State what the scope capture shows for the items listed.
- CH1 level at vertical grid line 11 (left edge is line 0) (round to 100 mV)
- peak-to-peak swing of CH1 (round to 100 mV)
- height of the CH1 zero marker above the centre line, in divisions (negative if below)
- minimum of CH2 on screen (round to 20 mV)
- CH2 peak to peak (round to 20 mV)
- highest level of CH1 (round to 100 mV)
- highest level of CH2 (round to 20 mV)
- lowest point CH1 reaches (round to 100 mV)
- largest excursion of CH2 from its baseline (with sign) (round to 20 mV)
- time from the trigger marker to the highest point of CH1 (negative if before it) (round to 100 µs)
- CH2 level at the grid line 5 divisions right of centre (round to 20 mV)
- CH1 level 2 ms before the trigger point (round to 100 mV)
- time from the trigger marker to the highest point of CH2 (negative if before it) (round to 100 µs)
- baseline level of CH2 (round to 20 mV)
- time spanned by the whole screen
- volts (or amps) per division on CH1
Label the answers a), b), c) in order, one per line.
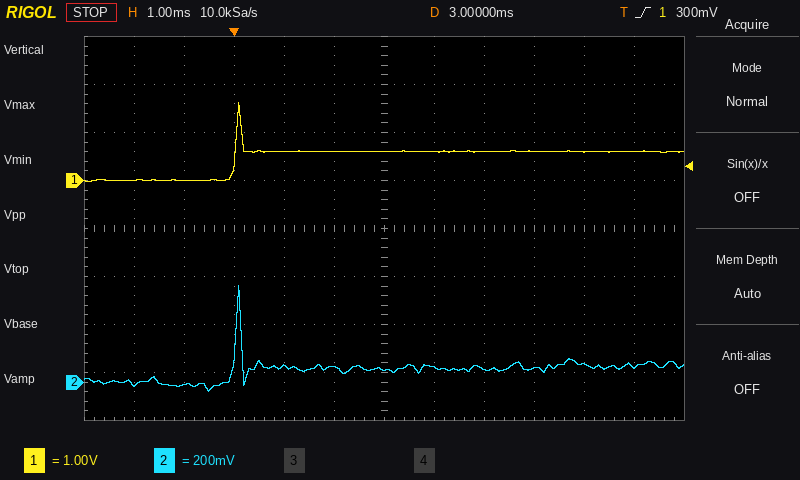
a) 600 mV
b) 1.6 V
c) +1.0 div
d) -40 mV
e) 440 mV
f) 1.6 V
g) 400 mV
h) 0.0 V
i) +340 mV
j) +100 µs
k) 60 mV
l) 0.0 V
m) +100 µs
n) 60 mV
o) 12 ms
p) 1 V
